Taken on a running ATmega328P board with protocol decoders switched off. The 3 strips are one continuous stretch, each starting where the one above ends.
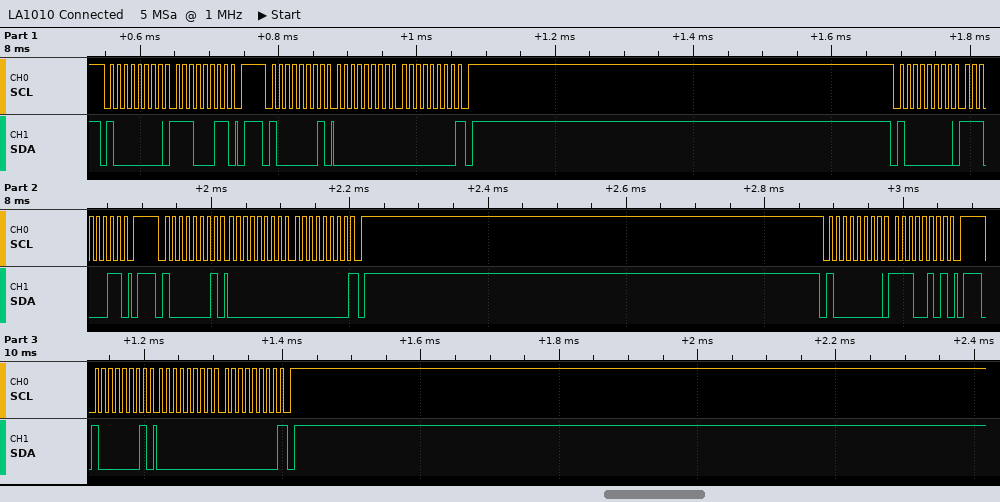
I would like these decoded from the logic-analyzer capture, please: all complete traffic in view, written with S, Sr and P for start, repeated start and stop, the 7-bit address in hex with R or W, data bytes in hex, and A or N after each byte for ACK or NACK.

S 40W A E3 A P S 40R A 00 A 00 N P S 40W A E3 A P S 40R A 00 A 00 N P S 40W A E5 A P S 40R A 00 A 00 N P
